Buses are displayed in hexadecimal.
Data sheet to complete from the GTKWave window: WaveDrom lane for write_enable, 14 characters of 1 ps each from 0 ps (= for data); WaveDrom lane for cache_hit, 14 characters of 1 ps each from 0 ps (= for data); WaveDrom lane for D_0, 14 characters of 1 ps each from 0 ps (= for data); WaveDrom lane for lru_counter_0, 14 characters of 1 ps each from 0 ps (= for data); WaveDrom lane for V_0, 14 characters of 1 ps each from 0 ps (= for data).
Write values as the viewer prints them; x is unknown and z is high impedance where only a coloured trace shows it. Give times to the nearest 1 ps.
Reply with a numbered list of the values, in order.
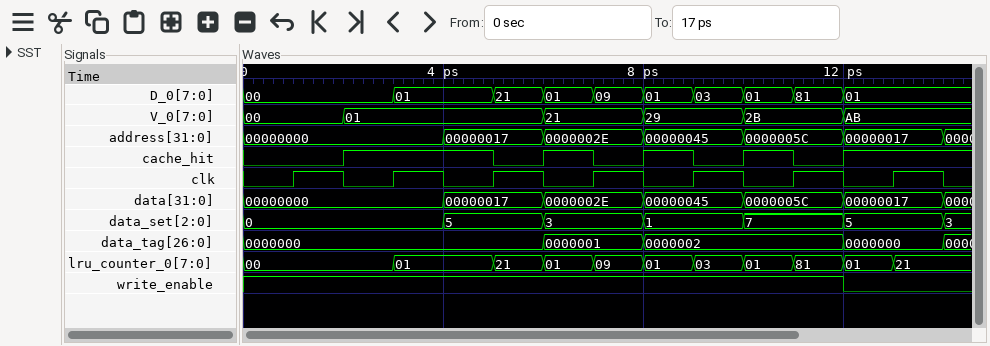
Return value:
1. {name: 'write_enable', wave: '1...........0.'}
2. {name: 'cache_hit', wave: '0.1..01010101.'}
3. {name: 'D_0', wave: '=..=.========.', data: '00 01 21 01 09 01 03 01 81 01'}
4. {name: 'lru_counter_0', wave: '=..=.=========', data: '00 01 21 01 09 01 03 01 81 01 21'}
5. {name: 'V_0', wave: '=.=...=.=.=.=.', data: '00 01 21 29 2B AB'}
